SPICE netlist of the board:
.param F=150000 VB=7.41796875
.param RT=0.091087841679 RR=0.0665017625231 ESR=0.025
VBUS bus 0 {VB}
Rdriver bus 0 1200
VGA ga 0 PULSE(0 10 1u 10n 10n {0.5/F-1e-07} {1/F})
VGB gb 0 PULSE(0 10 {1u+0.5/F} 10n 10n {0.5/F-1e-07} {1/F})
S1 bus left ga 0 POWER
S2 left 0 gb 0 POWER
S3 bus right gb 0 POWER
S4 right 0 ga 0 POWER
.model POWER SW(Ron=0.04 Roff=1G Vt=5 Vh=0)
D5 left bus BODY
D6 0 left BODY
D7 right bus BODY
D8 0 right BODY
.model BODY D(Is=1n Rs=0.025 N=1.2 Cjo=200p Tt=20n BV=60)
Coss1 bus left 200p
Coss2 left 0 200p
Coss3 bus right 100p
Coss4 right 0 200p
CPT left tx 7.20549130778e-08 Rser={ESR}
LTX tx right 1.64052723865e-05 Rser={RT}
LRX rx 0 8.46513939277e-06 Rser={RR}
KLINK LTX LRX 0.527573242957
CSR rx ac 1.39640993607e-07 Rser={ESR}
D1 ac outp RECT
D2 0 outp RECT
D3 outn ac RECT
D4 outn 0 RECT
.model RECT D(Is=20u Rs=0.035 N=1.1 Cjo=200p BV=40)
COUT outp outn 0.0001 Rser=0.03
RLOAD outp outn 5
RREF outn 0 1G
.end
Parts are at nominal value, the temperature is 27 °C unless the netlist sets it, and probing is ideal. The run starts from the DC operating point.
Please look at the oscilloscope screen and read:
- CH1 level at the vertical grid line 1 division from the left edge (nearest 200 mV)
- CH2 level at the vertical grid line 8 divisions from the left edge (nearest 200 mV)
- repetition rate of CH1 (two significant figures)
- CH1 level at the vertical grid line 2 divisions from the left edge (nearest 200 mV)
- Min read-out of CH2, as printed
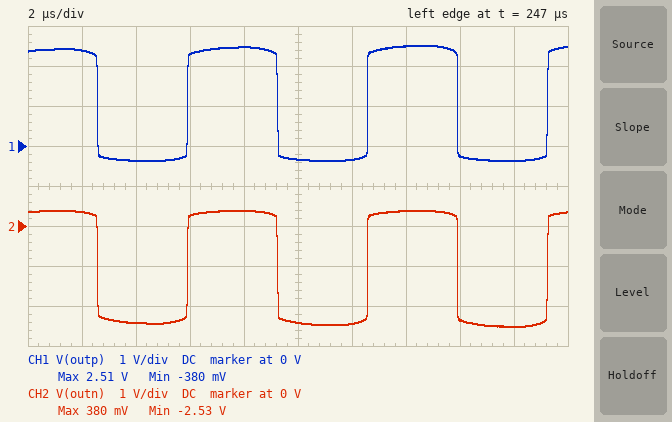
2.4 V
-2.4 V
150 kHz
-400 mV
-2.53 V
